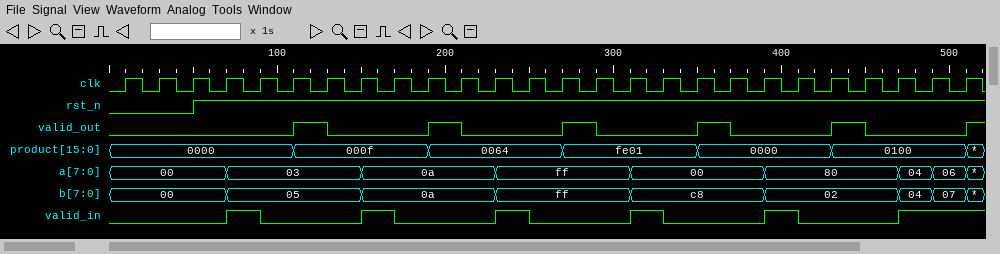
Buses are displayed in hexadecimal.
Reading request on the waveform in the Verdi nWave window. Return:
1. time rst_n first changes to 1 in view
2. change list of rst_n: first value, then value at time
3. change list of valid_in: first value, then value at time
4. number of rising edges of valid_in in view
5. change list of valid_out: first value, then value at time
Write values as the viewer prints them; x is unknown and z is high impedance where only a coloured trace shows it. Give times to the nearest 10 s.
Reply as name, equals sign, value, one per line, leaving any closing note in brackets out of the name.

time rst_n first changes to 1 in view = 50 s
change list of rst_n: first value, then value at time = 0, 1 at 50 s
change list of valid_in: first value, then value at time = 0, 1 at 70 s, 0 at 90 s, 1 at 150 s, 0 at 170 s, 1 at 230 s, 0 at 250 s, 1 at 310 s, 0 at 330 s, 1 at 390 s, 0 at 410 s, 1 at 470 s
number of rising edges of valid_in in view = 6
change list of valid_out: first value, then value at time = 0, 1 at 110 s, 0 at 130 s, 1 at 190 s, 0 at 210 s, 1 at 270 s, 0 at 290 s, 1 at 350 s, 0 at 370 s, 1 at 430 s, 0 at 450 s, 1 at 510 s
